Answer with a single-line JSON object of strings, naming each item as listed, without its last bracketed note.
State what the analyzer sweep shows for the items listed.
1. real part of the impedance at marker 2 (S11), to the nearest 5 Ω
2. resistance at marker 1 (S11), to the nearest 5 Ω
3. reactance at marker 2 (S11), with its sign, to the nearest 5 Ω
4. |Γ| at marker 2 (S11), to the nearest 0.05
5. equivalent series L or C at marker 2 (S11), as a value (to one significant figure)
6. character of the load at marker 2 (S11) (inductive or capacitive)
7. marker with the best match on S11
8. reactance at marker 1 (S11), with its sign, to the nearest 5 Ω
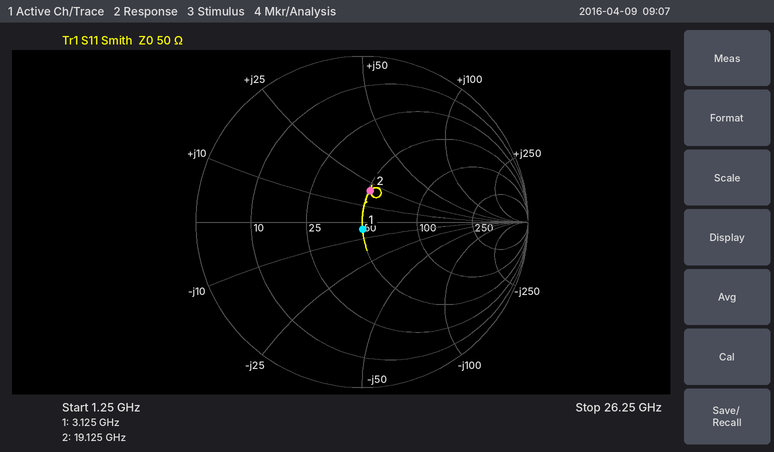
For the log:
{"real part of the impedance at marker 2 (S11), to the nearest 5 Ω": "50 Ω", "resistance at marker 1 (S11), to the nearest 5 Ω": "50 Ω", "reactance at marker 2 (S11), with its sign, to the nearest 5 Ω": "+20 Ω", "|Γ| at marker 2 (S11), to the nearest 0.05": "0.20", "equivalent series L or C at marker 2 (S11), as a value": "200 pH", "character of the load at marker 2 (S11)": "inductive", "marker with the best match on S11": "marker 1", "reactance at marker 1 (S11), with its sign, to the nearest 5 Ω": "-5 Ω"}
